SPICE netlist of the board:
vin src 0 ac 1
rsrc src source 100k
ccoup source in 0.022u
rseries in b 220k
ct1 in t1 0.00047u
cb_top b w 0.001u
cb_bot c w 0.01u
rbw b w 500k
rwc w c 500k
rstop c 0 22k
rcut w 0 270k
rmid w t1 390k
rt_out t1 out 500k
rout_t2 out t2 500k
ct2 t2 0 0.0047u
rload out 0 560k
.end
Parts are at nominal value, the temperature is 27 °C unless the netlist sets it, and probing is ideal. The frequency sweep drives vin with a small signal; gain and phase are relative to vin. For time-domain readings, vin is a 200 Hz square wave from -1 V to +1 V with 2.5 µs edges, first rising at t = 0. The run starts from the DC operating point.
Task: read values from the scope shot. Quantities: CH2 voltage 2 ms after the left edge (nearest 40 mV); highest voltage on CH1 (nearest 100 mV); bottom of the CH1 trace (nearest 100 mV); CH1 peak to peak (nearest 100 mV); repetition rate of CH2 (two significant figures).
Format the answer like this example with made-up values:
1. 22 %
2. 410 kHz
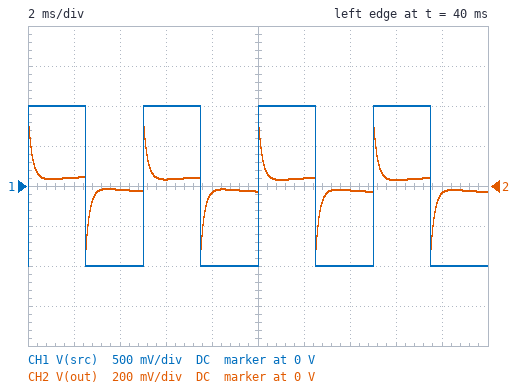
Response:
1. 40 mV
2. 1.0 V
3. -1.0 V
4. 2.0 V
5. 200 Hz
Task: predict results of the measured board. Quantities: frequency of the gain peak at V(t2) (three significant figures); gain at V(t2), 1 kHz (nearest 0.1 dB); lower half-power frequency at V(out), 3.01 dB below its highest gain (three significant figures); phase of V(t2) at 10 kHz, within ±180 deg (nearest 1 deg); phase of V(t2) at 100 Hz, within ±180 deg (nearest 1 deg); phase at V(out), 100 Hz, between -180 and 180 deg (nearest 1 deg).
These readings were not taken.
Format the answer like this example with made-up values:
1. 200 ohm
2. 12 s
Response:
1. 16.0 Hz
2. -40.1 dB
3. 894 Hz
4. -85 deg
5. -43 deg
6. 13 deg
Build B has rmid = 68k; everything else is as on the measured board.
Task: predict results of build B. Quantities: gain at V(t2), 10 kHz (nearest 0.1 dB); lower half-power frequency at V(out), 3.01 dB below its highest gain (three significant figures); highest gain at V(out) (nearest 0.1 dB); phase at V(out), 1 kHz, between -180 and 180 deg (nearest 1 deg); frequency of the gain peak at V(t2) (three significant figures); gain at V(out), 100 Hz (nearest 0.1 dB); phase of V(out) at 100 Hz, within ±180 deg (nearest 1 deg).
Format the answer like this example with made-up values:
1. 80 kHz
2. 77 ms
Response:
1. -60.9 dB
2. 2.43 kHz
3. -17.2 dB
4. 38 deg
5. 16.6 Hz
6. -27.7 dB
7. -15 deg
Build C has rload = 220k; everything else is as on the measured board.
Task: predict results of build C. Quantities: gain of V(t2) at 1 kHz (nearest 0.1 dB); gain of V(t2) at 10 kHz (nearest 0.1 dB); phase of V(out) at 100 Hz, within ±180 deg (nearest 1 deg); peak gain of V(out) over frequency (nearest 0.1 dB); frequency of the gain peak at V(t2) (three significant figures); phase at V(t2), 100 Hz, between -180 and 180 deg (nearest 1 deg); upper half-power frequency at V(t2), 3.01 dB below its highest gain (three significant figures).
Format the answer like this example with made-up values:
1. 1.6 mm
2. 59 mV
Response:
1. -43.8 dB
2. -61.0 dB
3. 19 deg
4. -17.6 dB
5. 17.9 Hz
6. -37 deg
7. 54.8 Hz
